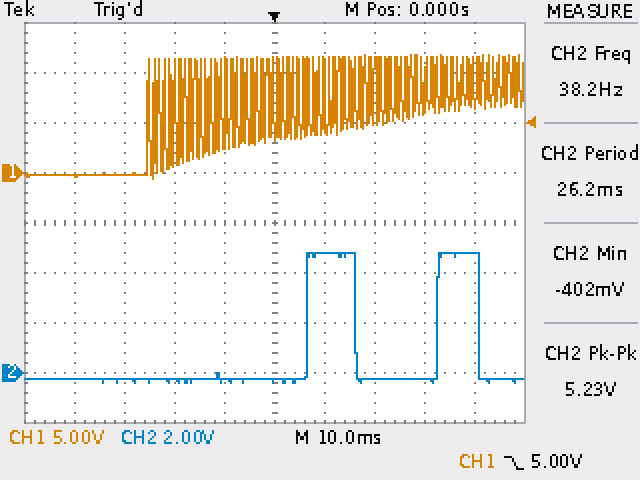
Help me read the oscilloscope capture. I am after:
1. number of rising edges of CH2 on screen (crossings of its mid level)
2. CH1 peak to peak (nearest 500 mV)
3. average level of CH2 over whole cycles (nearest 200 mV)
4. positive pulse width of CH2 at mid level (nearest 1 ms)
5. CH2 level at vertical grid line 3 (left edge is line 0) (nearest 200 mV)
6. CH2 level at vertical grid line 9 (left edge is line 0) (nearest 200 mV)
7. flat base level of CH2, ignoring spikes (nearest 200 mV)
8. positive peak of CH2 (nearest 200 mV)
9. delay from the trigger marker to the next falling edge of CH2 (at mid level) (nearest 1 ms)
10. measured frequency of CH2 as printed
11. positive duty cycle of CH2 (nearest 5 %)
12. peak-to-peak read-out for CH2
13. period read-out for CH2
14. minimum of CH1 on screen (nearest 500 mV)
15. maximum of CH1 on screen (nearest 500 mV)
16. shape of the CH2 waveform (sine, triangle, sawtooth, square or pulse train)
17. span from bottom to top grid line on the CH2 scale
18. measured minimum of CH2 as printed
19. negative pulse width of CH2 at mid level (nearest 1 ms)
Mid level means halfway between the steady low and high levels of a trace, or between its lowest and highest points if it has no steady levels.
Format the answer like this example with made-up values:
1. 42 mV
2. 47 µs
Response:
1. 2
2. 12.5 V
3. 1.6 V
4. 9 ms
5. -200 mV
6. 4.8 V
7. -200 mV
8. 4.8 V
9. 16 ms
10. 38.2 Hz
11. 35 %
12. 5.23 V
13. 26.2 ms
14. -500 mV
15. 12.0 V
16. pulse train
17. 16 V
18. -402 mV
19. 17 ms
